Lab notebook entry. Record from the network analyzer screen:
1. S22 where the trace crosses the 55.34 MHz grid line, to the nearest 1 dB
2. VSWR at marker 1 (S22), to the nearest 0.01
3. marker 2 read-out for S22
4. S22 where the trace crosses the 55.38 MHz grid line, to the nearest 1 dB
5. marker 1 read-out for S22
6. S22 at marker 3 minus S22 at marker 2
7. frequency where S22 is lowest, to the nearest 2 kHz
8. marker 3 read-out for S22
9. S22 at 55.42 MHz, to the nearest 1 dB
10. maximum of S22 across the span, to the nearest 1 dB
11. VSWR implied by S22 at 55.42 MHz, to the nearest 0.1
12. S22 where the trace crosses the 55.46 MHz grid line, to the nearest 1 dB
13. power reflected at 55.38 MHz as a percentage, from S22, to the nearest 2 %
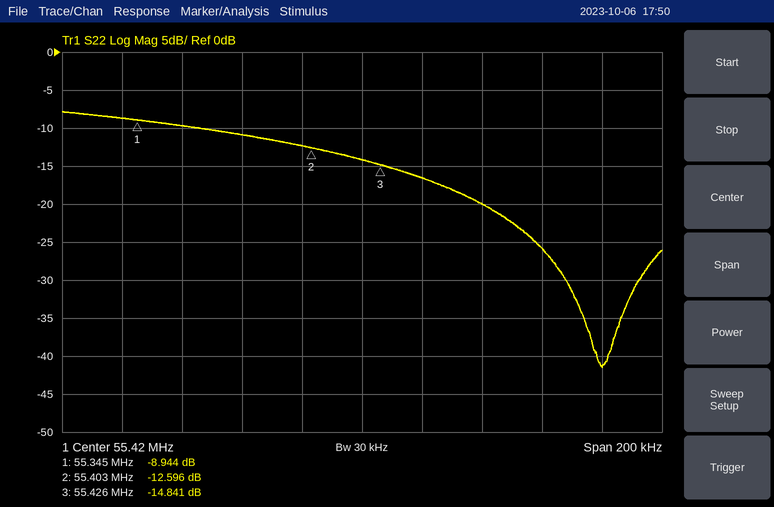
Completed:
-9 dB
2.11
-12.596 dB
-11 dB
-8.944 dB
-2.245 dB
55.500 MHz
-14.841 dB
-14 dB
-8 dB
1.5
-20 dB
8 %
